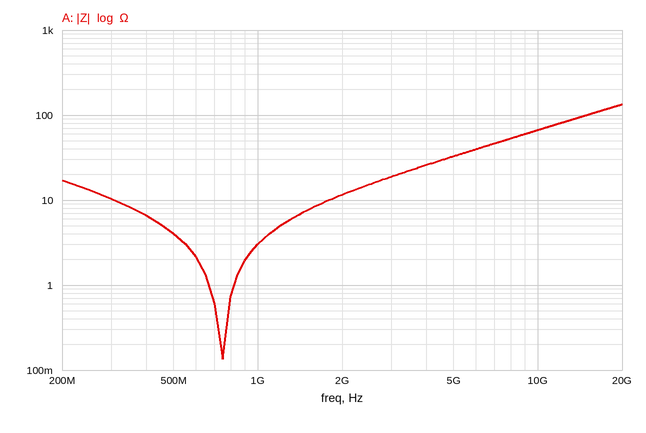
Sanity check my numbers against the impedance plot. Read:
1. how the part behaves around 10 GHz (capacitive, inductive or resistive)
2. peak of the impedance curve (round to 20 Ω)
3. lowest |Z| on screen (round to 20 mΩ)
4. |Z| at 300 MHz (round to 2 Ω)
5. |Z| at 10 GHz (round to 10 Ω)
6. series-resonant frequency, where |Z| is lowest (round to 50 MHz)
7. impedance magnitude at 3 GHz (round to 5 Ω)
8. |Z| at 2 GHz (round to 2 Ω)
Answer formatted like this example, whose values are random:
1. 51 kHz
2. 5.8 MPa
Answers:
1. inductive
2. 140 Ω
3. 140 mΩ
4. 10 Ω
5. 70 Ω
6. 750 MHz
7. 20 Ω
8. 12 Ω
